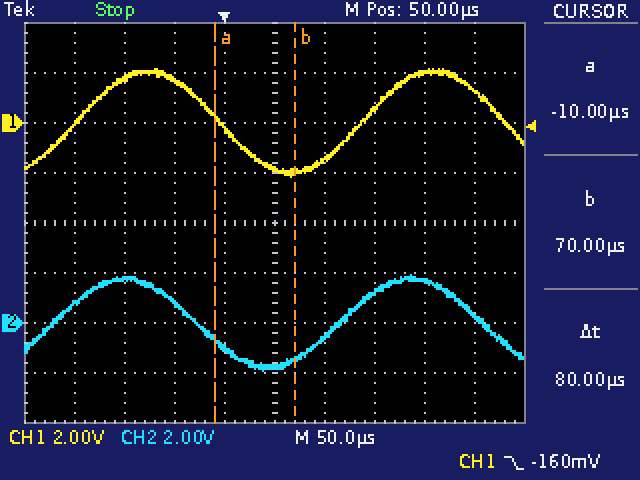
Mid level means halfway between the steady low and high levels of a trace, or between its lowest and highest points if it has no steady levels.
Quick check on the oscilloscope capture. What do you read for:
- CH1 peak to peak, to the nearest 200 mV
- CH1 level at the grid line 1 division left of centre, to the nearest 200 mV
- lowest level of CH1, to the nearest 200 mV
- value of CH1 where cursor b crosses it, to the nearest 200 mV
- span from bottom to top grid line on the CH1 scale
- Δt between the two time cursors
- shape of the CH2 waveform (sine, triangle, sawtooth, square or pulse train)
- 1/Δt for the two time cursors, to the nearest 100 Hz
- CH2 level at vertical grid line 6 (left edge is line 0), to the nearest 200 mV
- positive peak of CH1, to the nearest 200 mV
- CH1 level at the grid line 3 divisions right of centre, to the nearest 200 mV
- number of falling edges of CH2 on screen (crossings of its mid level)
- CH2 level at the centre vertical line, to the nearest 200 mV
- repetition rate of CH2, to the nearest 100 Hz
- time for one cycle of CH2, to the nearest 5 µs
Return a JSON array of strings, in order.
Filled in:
["4.4 V", "-200 mV", "-2.2 V", "-2.0 V", "16 V", "80 µs", "sine", "12.5 kHz", "-600 mV", "2.2 V", "2.0 V", "2", "-1.8 V", "3.5 kHz", "285 µs"]
